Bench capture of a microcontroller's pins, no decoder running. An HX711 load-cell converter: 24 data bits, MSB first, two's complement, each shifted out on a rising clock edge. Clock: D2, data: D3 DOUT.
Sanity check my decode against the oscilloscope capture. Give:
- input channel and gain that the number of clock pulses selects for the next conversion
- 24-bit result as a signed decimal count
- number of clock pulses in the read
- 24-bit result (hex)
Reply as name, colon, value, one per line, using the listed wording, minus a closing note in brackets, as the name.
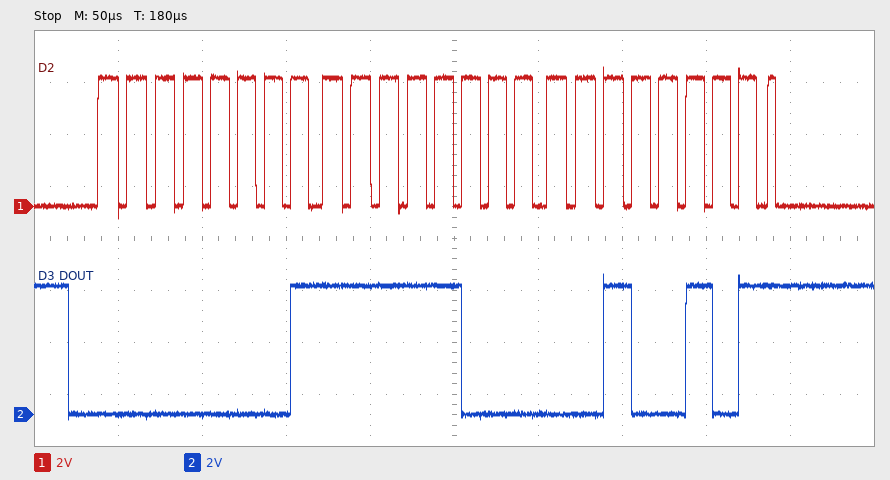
input channel and gain that the number of clock pulses selects for the next conversion: channel A, gain 128
24-bit result as a signed decimal count: 129061
number of clock pulses in the read: 25
24-bit result: 0x01F825
